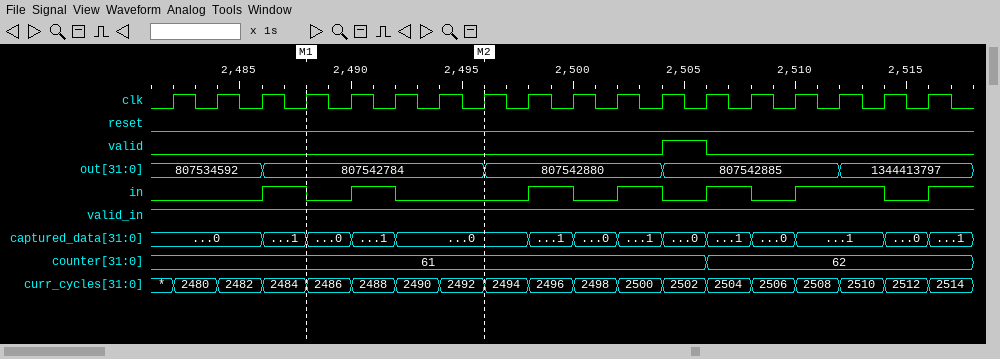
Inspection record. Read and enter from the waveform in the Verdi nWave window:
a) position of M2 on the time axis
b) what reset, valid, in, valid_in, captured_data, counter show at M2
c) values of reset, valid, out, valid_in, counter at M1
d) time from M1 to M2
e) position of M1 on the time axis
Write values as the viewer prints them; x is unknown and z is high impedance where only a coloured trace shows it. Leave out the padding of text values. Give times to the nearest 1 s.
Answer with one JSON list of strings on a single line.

["2496 s", "reset=0, valid=0, in=0, valid_in=1, captured_data=0, counter=61", "reset=0, valid=0, out=807542784, valid_in=1, counter=61", "8 s", "2488 s"]
